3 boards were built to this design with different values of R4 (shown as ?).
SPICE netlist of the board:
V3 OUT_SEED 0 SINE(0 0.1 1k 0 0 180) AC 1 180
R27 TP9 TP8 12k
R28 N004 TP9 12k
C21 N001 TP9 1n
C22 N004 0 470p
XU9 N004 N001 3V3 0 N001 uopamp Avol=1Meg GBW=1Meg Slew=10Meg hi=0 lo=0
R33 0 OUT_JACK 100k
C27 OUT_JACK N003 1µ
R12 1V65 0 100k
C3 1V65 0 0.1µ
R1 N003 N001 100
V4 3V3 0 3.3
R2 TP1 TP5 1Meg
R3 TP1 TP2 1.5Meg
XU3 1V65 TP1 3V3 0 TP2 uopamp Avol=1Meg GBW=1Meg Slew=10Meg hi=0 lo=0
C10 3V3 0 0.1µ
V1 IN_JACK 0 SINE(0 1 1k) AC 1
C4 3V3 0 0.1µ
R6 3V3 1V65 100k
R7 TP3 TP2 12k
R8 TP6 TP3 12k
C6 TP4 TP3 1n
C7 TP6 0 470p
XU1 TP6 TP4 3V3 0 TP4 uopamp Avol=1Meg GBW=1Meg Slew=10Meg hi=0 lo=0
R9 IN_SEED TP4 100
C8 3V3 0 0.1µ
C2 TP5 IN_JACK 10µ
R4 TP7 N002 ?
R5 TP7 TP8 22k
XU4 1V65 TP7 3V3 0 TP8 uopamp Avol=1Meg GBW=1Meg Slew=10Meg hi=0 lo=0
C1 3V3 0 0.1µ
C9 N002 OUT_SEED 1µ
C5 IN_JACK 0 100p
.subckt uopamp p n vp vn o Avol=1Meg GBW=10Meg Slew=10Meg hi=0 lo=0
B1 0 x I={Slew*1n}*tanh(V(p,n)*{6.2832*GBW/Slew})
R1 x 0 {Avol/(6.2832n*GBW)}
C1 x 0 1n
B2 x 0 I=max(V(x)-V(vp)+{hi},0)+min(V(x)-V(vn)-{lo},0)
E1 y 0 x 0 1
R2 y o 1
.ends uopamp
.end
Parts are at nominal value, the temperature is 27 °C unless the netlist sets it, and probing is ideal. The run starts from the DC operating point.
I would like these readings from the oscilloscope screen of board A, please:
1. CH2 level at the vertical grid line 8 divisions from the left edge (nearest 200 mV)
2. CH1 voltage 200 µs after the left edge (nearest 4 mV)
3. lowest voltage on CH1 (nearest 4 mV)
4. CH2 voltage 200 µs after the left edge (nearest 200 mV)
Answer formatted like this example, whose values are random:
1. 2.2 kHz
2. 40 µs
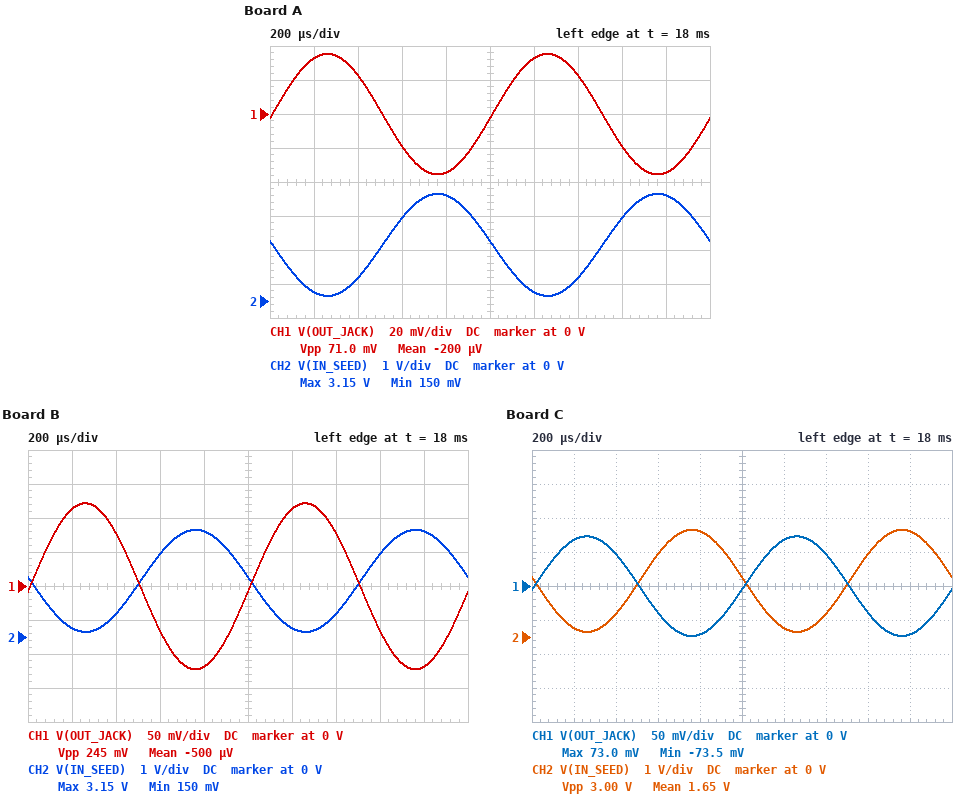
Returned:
1. 2.4 V
2. 32 mV
3. -36 mV
4. 200 mV
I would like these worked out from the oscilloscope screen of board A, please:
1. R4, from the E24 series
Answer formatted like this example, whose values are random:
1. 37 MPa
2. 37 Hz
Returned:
1. 62 kΩ
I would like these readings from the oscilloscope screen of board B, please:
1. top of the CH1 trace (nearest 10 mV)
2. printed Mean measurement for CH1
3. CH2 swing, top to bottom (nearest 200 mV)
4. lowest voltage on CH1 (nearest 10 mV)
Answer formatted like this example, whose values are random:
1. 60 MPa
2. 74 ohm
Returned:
1. 120 mV
2. -500 µV
3. 3.0 V
4. -120 mV
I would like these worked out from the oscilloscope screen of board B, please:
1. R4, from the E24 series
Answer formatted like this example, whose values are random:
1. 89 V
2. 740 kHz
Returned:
1. 18 kΩ
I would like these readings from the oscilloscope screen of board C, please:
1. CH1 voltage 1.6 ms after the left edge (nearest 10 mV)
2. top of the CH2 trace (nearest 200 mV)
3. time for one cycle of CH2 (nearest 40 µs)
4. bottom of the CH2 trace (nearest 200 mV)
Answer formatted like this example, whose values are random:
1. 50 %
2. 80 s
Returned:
1. -40 mV
2. 3.2 V
3. 1.00 ms
4. 200 mV
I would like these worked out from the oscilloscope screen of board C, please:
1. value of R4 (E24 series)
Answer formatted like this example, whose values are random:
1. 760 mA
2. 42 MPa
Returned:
1. 30 kΩ
